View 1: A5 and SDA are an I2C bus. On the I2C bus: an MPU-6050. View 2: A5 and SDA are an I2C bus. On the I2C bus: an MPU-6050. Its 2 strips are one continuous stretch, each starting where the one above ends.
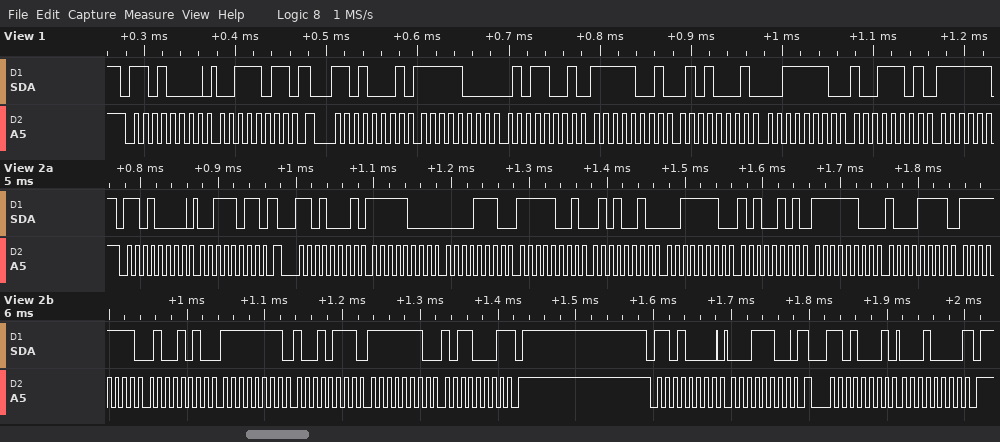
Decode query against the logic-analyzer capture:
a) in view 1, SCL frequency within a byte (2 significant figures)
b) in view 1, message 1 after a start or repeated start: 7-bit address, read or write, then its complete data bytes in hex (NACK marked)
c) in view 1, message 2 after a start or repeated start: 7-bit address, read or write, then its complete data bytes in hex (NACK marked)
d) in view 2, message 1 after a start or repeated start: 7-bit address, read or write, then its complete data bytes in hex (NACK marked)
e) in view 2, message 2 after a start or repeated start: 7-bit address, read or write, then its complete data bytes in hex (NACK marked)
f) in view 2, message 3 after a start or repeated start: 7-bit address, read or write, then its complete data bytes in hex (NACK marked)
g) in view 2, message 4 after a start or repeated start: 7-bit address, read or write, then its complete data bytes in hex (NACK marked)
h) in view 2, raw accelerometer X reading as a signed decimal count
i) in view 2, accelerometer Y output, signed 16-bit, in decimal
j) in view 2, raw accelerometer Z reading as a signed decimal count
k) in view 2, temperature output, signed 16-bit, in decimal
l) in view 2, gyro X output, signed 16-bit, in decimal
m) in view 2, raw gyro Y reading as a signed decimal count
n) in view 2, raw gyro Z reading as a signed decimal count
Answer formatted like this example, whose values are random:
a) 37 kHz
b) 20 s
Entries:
a) 100 kHz
b) 0x68 write: 3B
c) 0x68 read: F8 59 F9 51 3E 9D
d) 0x68 write: 3B
e) 0x68 read: F8 0E F9 52 3E A5 FC 8F FF 4A FF 97 FE B1 NACK
f) 0x68 write: 1C
g) 0x68 read: 10 NACK
h) -2034
i) -1710
j) 16037
k) -881
l) -182
m) -105
n) -335
